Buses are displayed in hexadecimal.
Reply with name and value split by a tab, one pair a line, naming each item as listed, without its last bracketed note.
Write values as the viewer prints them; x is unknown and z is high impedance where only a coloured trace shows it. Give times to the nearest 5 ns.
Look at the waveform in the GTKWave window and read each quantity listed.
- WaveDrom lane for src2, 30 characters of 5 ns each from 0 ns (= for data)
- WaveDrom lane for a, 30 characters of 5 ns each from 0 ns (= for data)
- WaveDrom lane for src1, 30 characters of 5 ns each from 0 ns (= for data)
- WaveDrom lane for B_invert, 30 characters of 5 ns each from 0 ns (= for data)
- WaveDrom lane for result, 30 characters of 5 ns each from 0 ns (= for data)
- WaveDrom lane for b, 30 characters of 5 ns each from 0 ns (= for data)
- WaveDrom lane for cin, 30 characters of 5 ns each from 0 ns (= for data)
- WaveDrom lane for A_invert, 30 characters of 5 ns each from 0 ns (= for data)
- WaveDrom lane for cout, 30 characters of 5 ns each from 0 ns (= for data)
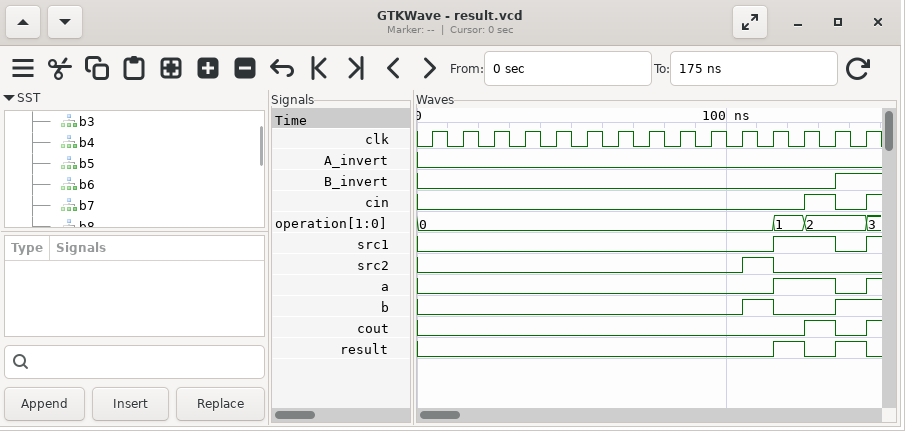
WaveDrom lane for src2, 30 characters of 5 ns each from 0 ns	{name: 'src2', wave: '0....................1.0......'}
WaveDrom lane for a, 30 characters of 5 ns each from 0 ns	{name: 'a', wave: '0......................1...0.1'}
WaveDrom lane for src1, 30 characters of 5 ns each from 0 ns	{name: 'src1', wave: '0......................1...0.1'}
WaveDrom lane for B_invert, 30 characters of 5 ns each from 0 ns	{name: 'B_invert', wave: '0..........................1..'}
WaveDrom lane for result, 30 characters of 5 ns each from 0 ns	{name: 'result', wave: '0......................1.0.1.0'}
WaveDrom lane for b, 30 characters of 5 ns each from 0 ns	{name: 'b', wave: '0....................1.0...1..'}
WaveDrom lane for cin, 30 characters of 5 ns each from 0 ns	{name: 'cin', wave: '0........................1.0.1'}
WaveDrom lane for A_invert, 30 characters of 5 ns each from 0 ns	{name: 'A_invert', wave: '0.............................'}
WaveDrom lane for cout, 30 characters of 5 ns each from 0 ns	{name: 'cout', wave: '0........................1.0.1'}
